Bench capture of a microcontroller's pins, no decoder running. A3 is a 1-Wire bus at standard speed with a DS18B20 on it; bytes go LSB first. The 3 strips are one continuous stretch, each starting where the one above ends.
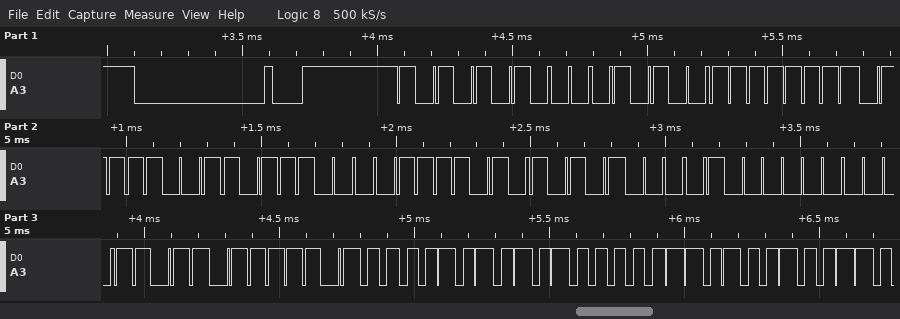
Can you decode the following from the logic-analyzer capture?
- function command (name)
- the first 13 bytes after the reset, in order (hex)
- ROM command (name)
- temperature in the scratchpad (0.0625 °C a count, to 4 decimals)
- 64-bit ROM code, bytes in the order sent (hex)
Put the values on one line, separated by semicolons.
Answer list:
Read Scratchpad; 55 28 FF 9E 1D 5E 15 02 D8 BE 50 05 4B; Match ROM; 85.0000 °C; 28 FF 9E 1D 5E 15 02 D8
